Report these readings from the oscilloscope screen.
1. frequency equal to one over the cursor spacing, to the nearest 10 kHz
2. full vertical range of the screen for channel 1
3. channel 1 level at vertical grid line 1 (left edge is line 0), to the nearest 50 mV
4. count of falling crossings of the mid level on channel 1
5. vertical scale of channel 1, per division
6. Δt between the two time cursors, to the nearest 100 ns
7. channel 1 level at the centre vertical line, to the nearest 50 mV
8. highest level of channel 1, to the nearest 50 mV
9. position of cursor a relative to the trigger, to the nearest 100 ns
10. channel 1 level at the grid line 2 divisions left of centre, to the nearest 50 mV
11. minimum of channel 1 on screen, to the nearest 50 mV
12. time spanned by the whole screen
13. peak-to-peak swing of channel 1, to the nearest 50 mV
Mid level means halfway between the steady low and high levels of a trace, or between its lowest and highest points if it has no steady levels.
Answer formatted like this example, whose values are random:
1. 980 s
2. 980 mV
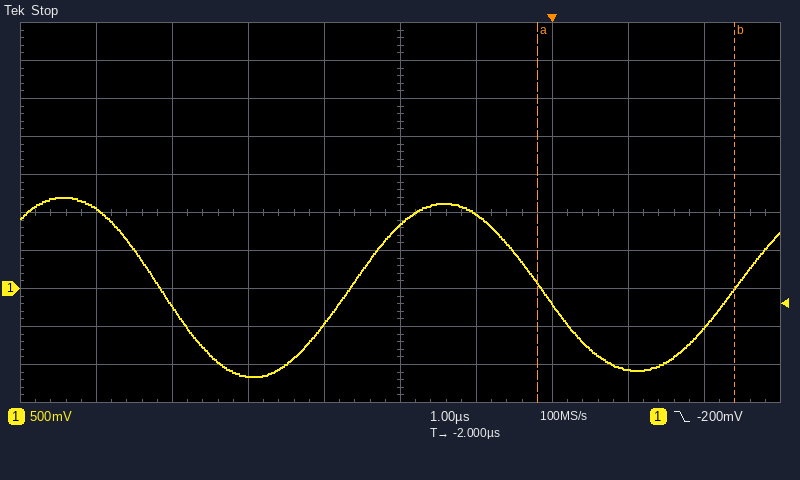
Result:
1. 380 kHz
2. 5 V
3. 1.05 V
4. 2
5. 500 mV
6. 2.6 µs
7. 850 mV
8. 1.20 V
9. -200 ns
10. -1.15 V
11. -1.15 V
12. 10 µs
13. 2.35 V
